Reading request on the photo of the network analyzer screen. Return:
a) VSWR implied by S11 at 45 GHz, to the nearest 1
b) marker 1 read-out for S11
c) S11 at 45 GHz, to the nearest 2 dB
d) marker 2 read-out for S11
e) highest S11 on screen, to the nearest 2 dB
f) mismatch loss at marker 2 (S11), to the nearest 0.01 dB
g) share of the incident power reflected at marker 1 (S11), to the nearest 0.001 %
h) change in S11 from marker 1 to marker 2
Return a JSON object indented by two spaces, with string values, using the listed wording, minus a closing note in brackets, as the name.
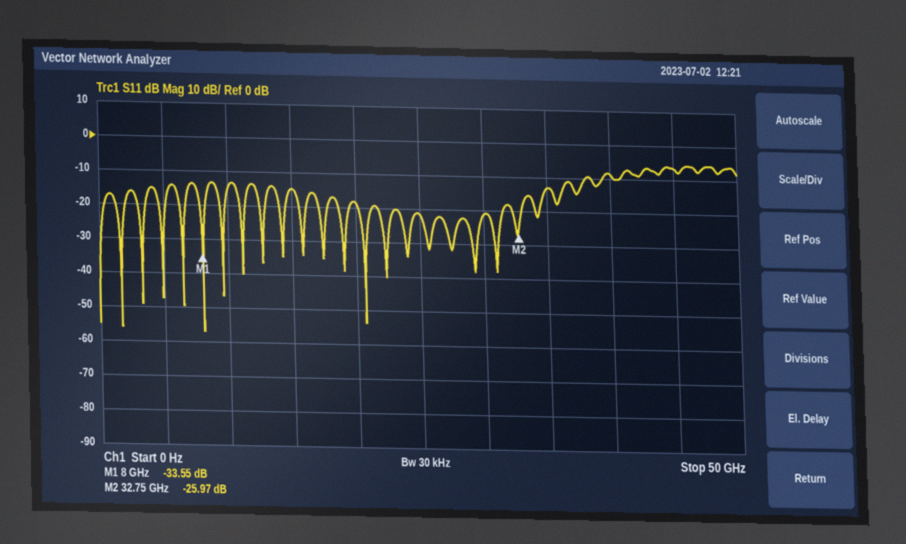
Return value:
{
  "VSWR implied by S11 at 45 GHz, to the nearest 1": "3",
  "marker 1 read-out for S11": "-33.55 dB",
  "S11 at 45 GHz, to the nearest 2 dB": "-6 dB",
  "marker 2 read-out for S11": "-25.97 dB",
  "highest S11 on screen, to the nearest 2 dB": "-6 dB",
  "mismatch loss at marker 2 (S11), to the nearest 0.01 dB": "0.01 dB",
  "share of the incident power reflected at marker 1 (S11), to the nearest 0.001 %": "0.044 %",
  "change in S11 from marker 1 to marker 2": "7.58 dB"
}
